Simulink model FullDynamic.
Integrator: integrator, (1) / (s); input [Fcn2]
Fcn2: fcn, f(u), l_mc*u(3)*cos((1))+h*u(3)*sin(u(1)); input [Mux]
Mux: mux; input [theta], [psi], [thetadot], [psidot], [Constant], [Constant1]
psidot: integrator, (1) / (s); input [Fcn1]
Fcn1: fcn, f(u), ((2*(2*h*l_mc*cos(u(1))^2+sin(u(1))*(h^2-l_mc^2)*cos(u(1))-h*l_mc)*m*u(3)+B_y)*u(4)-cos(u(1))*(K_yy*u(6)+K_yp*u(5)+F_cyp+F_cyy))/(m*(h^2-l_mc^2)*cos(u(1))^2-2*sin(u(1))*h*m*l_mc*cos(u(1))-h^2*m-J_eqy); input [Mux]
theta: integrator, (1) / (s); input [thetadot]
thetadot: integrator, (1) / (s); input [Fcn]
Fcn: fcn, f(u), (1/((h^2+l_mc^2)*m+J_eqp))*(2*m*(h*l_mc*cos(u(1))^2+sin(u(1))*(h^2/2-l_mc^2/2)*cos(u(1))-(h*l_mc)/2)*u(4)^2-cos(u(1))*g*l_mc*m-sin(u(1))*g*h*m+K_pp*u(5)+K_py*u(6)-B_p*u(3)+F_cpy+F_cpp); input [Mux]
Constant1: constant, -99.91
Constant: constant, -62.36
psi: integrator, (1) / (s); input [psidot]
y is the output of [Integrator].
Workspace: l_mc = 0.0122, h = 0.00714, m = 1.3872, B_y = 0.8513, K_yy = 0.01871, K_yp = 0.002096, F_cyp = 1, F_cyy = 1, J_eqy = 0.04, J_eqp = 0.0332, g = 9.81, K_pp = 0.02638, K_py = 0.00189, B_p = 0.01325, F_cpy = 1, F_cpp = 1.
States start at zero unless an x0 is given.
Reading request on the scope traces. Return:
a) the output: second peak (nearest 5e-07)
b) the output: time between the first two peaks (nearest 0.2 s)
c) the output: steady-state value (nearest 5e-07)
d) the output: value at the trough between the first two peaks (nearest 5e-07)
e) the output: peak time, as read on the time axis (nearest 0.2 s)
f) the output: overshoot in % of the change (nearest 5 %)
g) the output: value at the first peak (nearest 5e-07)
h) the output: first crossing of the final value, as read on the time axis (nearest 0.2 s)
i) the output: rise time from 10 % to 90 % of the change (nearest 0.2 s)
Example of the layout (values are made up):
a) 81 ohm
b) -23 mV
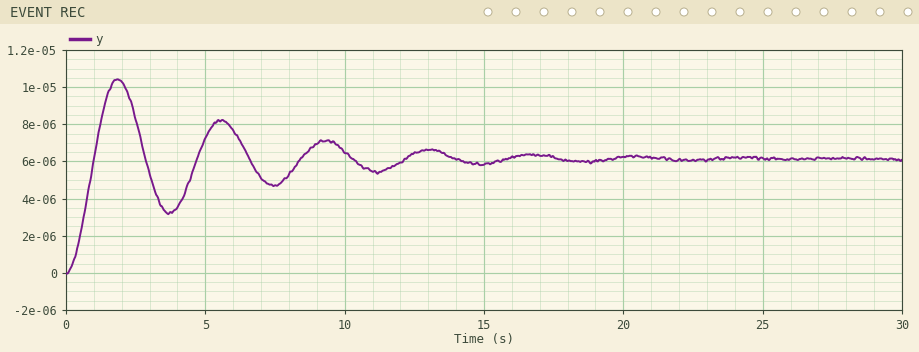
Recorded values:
a) 0.0000080
b) 3.8 s
c) 0.0000060
d) 0.0000030
e) 1.8 s
f) 70 %
g) 0.0000105
h) 1.0 s
i) 0.6 s
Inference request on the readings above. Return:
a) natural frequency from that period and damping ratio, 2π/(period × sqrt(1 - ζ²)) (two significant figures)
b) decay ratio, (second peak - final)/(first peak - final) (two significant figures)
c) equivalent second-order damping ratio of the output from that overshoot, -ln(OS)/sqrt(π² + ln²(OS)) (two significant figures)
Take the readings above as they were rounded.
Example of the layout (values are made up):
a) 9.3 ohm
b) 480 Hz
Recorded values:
a) 1.7 rad/s
b) 0.44
c) 0.11
